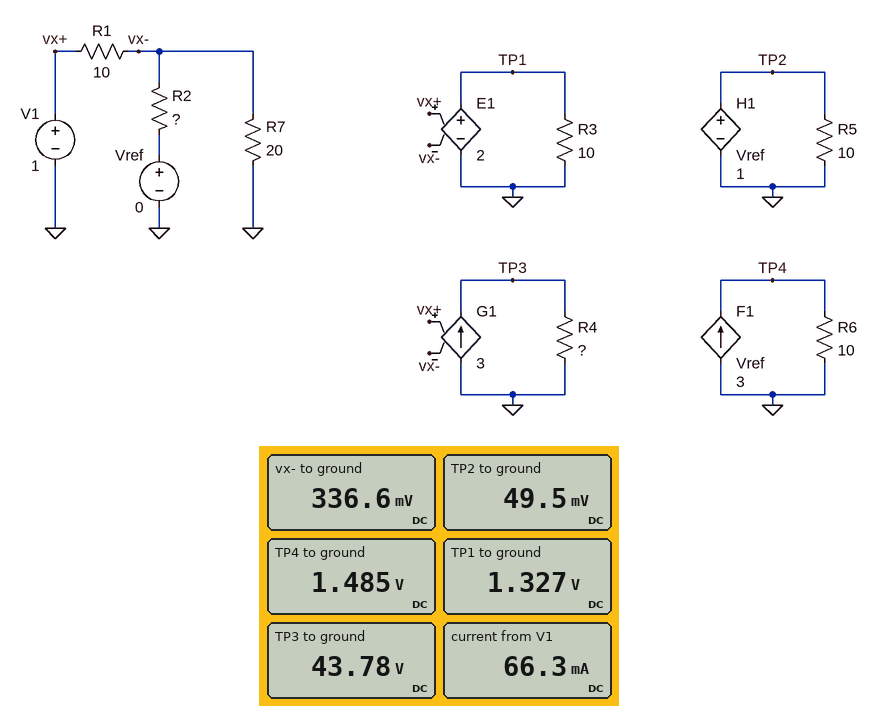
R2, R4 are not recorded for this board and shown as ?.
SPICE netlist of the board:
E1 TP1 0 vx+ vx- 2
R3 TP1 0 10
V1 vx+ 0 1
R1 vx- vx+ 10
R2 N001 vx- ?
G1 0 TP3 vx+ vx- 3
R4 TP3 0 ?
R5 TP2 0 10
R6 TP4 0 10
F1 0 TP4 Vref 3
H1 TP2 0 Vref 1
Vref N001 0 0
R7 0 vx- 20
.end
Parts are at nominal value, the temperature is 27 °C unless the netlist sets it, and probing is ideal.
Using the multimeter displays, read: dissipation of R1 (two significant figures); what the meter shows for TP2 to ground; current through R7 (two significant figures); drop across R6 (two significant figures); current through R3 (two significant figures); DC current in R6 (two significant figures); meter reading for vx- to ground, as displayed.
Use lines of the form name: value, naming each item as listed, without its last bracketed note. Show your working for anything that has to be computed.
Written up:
dissipation of R1: (1 V - 336.6 mV)^2 / 10 Ω = 44 mW
what the meter shows for TP2 to ground: 49.5 mV
current through R7: (336.6 mV) / 20 Ω = 17 mA
drop across R6: 1.485 V = 1.5 V
current through R3: (1.327 V) / 10 Ω = 130 mA
DC current in R6: (1.485 V) / 10 Ω = 150 mA
meter reading for vx- to ground, as displayed: 336.6 mV
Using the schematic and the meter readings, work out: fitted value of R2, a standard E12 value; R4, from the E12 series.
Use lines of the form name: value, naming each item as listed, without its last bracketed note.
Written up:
fitted value of R2, a standard E12 value: 6.8 Ω
R4, from the E12 series: 22 Ω
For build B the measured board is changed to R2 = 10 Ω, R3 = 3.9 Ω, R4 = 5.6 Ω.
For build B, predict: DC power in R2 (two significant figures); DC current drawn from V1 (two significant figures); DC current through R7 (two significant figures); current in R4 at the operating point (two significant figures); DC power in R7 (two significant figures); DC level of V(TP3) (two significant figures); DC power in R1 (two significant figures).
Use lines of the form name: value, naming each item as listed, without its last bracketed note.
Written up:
DC power in R2: 16 mW
DC current drawn from V1: 60 mA
DC current through R7: 20 mA
current in R4 at the operating point: 1.8 A
DC power in R7: 8.0 mW
DC level of V(TP3): 10 V
DC power in R1: 36 mW
